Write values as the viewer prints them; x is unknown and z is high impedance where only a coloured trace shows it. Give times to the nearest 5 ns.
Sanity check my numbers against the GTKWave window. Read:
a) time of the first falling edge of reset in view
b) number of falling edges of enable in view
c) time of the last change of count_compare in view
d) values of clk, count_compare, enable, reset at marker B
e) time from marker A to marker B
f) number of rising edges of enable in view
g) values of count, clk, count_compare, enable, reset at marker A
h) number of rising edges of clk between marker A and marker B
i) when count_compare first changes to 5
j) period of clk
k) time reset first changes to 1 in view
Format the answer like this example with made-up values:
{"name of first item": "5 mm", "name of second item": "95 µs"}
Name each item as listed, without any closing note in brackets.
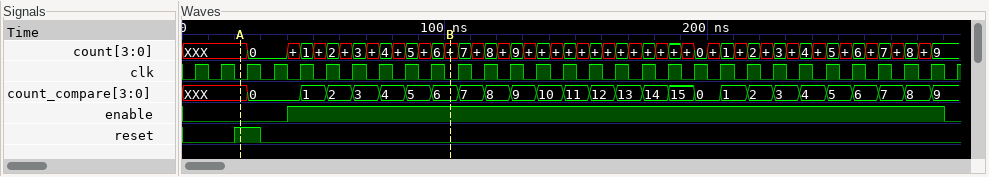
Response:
{"time of the first falling edge of reset in view": "30 ns", "number of falling edges of enable in view": "1", "time of the last change of count_compare in view": "285 ns", "values of clk, count_compare, enable, reset at marker B": "clk=0, count_compare=6, enable=1, reset=0", "time from marker A to marker B": "80 ns", "number of rising edges of enable in view": "1", "values of count, clk, count_compare, enable, reset at marker A": "count=XXX, clk=0, count_compare=XXX, enable=0, reset=1", "number of rising edges of clk between marker A and marker B": "8", "when count_compare first changes to 5": "85 ns", "period of clk": "10 ns", "time reset first changes to 1 in view": "20 ns"}
